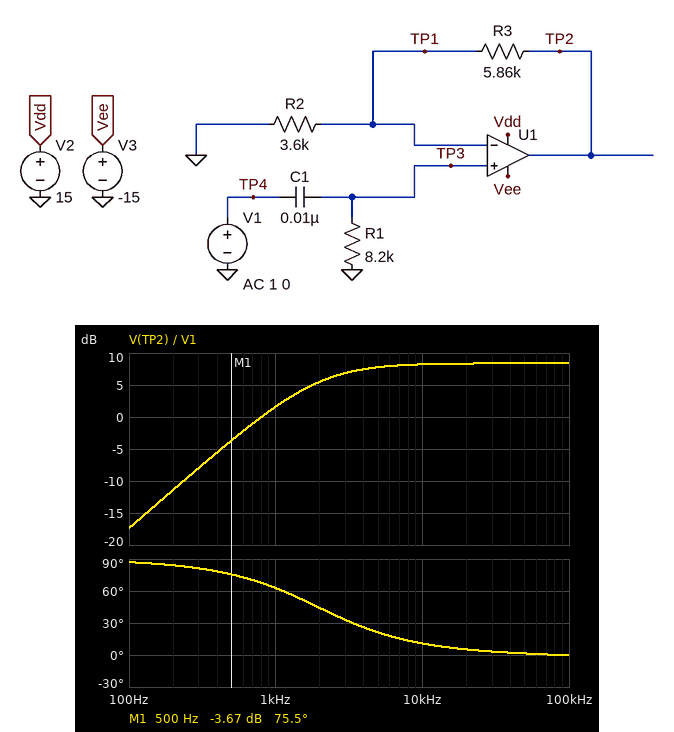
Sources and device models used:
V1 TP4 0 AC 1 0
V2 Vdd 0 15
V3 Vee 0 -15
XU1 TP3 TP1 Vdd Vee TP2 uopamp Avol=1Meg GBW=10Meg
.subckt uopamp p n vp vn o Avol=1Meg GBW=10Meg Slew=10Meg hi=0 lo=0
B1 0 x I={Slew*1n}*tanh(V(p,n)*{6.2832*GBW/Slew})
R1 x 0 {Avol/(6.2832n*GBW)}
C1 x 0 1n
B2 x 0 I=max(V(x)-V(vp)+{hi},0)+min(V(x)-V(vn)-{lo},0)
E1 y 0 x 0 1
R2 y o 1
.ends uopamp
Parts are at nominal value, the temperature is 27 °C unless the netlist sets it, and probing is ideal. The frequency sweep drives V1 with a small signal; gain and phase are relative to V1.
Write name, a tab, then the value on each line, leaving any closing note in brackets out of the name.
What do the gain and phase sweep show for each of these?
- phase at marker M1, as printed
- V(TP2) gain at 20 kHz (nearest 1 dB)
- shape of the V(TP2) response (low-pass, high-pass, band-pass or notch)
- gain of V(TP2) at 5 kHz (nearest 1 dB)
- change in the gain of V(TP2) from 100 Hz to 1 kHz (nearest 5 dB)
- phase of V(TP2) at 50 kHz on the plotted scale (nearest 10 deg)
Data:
phase at marker M1, as printed	75.5 deg
V(TP2) gain at 20 kHz	8 dB
shape of the V(TP2) response	high-pass
gain of V(TP2) at 5 kHz	8 dB
change in the gain of V(TP2) from 100 Hz to 1 kHz	20 dB
phase of V(TP2) at 50 kHz on the plotted scale	0 deg
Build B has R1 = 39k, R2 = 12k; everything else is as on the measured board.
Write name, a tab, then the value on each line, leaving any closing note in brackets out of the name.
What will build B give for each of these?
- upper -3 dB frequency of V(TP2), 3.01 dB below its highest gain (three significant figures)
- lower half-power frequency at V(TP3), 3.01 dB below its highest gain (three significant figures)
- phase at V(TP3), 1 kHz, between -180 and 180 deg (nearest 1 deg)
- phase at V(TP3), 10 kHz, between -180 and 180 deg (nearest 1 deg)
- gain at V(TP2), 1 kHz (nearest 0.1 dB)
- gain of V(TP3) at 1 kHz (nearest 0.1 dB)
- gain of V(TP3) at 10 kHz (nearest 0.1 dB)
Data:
upper -3 dB frequency of V(TP2), 3.01 dB below its highest gain	6.72 MHz
lower half-power frequency at V(TP3), 3.01 dB below its highest gain	408 Hz
phase at V(TP3), 1 kHz, between -180 and 180 deg	22 deg
phase at V(TP3), 10 kHz, between -180 and 180 deg	2 deg
gain at V(TP2), 1 kHz	2.8 dB
gain of V(TP3) at 1 kHz	-0.7 dB
gain of V(TP3) at 10 kHz	0 dB
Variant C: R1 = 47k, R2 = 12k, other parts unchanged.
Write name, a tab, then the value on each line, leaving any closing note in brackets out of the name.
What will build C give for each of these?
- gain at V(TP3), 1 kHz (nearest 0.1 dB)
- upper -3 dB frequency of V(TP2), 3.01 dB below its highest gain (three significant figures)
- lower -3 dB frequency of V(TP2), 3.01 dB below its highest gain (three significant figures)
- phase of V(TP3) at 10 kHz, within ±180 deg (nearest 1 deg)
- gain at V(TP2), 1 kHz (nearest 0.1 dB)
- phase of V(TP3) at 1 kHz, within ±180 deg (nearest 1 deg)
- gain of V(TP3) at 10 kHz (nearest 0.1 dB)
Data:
gain at V(TP3), 1 kHz	-0.5 dB
upper -3 dB frequency of V(TP2), 3.01 dB below its highest gain	6.72 MHz
lower -3 dB frequency of V(TP2), 3.01 dB below its highest gain	339 Hz
phase of V(TP3) at 10 kHz, within ±180 deg	2 deg
gain at V(TP2), 1 kHz	3.0 dB
phase of V(TP3) at 1 kHz, within ±180 deg	19 deg
gain of V(TP3) at 10 kHz	0 dB
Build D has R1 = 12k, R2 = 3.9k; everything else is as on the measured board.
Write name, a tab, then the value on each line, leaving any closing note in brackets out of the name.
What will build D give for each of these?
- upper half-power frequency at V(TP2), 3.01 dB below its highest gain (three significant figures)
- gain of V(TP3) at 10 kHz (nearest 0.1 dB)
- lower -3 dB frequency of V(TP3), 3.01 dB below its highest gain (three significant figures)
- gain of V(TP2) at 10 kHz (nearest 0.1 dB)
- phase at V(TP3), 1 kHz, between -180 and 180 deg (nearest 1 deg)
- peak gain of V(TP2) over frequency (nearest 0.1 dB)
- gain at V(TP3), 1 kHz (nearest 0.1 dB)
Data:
upper half-power frequency at V(TP2), 3.01 dB below its highest gain	4.00 MHz
gain of V(TP3) at 10 kHz	-0.1 dB
lower -3 dB frequency of V(TP3), 3.01 dB below its highest gain	1.33 kHz
gain of V(TP2) at 10 kHz	7.9 dB
phase at V(TP3), 1 kHz, between -180 and 180 deg	53 deg
peak gain of V(TP2) over frequency	8.0 dB
gain at V(TP3), 1 kHz	-4.4 dB
